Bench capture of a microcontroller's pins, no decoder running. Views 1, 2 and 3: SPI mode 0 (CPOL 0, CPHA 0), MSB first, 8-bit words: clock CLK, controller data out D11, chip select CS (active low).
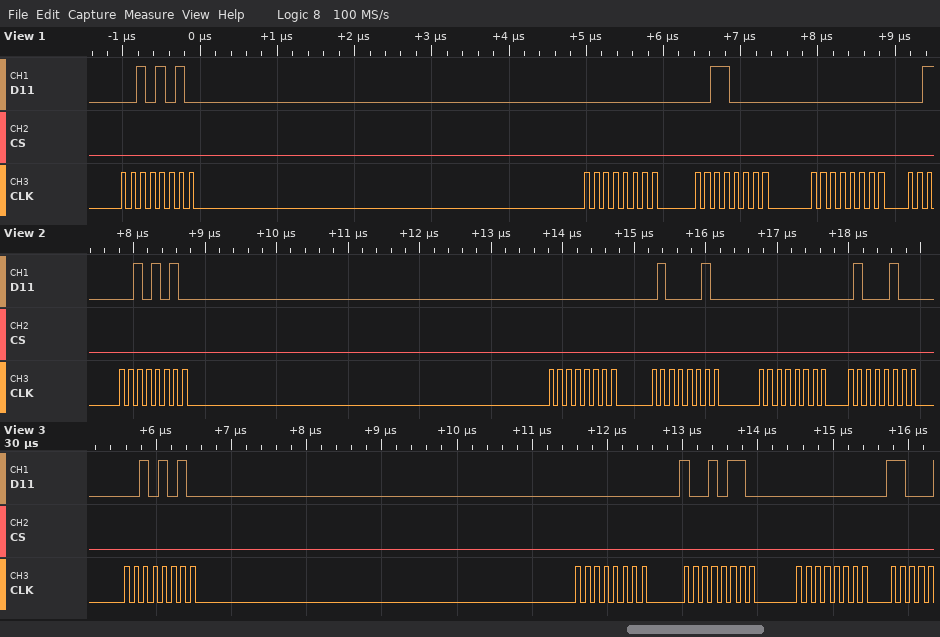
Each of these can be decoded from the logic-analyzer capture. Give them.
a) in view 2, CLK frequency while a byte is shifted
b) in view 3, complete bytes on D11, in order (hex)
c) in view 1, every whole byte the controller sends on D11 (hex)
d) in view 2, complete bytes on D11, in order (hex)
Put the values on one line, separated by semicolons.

8 MHz; 2A 00 96 00; 0x2A 0x00 0x30 0x00; 0x2A 0x00 0x42 0x00 0x44
